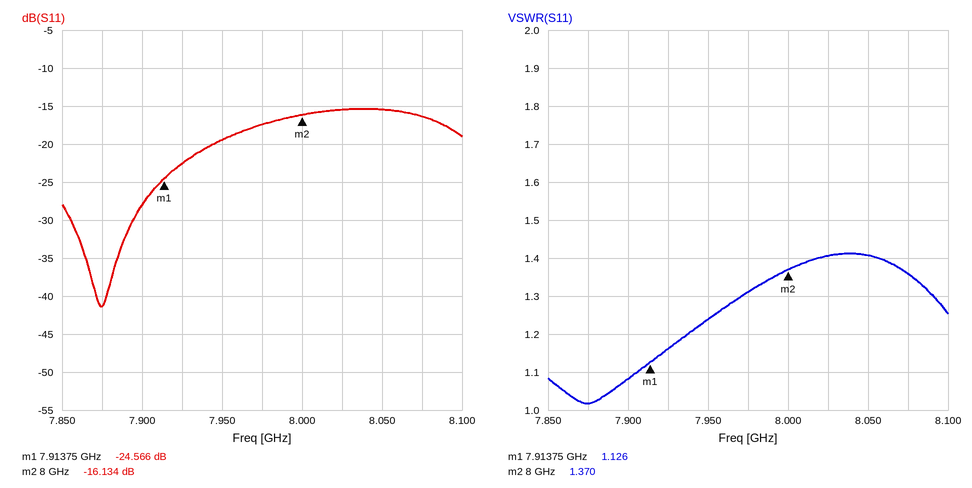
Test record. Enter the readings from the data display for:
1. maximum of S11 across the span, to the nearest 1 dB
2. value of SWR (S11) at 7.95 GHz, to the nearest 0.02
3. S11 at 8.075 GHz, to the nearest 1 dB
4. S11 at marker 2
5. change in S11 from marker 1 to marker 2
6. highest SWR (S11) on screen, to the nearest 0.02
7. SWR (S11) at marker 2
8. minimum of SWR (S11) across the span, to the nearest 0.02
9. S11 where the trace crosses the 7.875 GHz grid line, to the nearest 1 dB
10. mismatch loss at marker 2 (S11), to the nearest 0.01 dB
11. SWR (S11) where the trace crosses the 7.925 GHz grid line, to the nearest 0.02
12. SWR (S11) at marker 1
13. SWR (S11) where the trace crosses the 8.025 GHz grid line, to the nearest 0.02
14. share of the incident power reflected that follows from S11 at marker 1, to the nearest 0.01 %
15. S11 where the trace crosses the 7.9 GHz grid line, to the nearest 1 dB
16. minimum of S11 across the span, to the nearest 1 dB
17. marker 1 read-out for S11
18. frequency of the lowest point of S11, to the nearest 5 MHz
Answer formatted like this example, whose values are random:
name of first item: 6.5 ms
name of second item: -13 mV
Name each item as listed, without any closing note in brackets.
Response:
maximum of S11 across the span, to the nearest 1 dB: -15 dB
value of SWR (S11) at 7.95 GHz, to the nearest 0.02: 1.24
S11 at 8.075 GHz, to the nearest 1 dB: -16 dB
S11 at marker 2: -16.134 dB
change in S11 from marker 1 to marker 2: 8.432 dB
highest SWR (S11) on screen, to the nearest 0.02: 1.42
SWR (S11) at marker 2: 1.370
minimum of SWR (S11) across the span, to the nearest 0.02: 1.02
S11 where the trace crosses the 7.875 GHz grid line, to the nearest 1 dB: -41 dB
mismatch loss at marker 2 (S11), to the nearest 0.01 dB: 0.11 dB
SWR (S11) where the trace crosses the 7.925 GHz grid line, to the nearest 0.02: 1.16
SWR (S11) at marker 1: 1.126
SWR (S11) where the trace crosses the 8.025 GHz grid line, to the nearest 0.02: 1.40
share of the incident power reflected that follows from S11 at marker 1, to the nearest 0.01 %: 0.35 %
S11 where the trace crosses the 7.9 GHz grid line, to the nearest 1 dB: -28 dB
minimum of S11 across the span, to the nearest 1 dB: -41 dB
marker 1 read-out for S11: -24.566 dB
frequency of the lowest point of S11, to the nearest 5 MHz: 7.875 GHz
